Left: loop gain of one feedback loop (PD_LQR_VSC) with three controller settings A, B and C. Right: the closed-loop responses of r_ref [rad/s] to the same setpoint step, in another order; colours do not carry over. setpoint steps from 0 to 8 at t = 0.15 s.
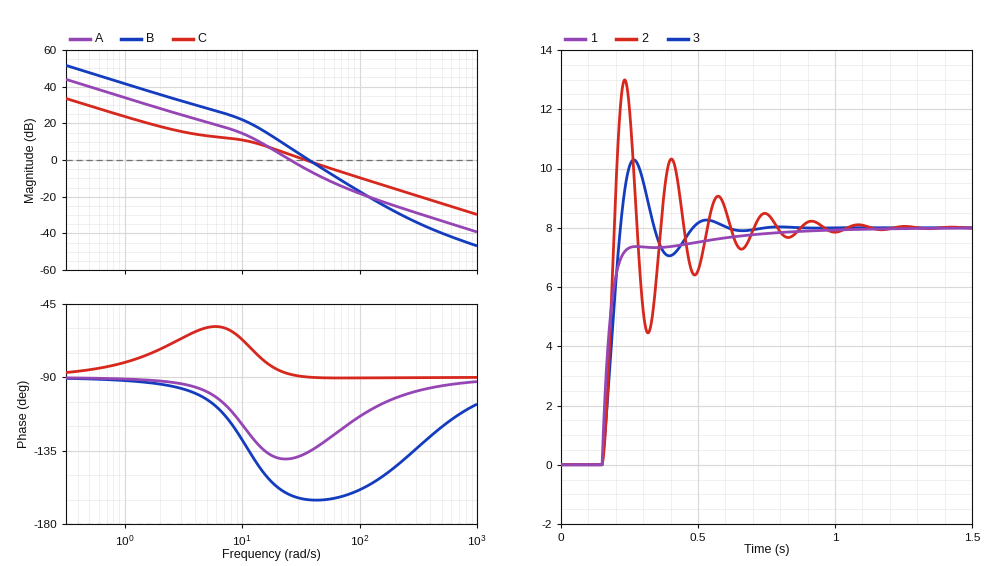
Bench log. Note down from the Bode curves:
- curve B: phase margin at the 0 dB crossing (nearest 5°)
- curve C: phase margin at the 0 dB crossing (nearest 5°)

15°
90°
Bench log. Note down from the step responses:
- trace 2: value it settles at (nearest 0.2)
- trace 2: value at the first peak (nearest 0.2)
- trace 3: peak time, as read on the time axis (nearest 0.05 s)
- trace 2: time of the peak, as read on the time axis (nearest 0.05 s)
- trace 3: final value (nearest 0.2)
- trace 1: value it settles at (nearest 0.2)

8.0
13.0
0.25 s
0.25 s
8.0
8.0
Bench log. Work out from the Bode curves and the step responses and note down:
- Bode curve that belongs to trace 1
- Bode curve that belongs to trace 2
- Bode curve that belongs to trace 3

C
B
A
